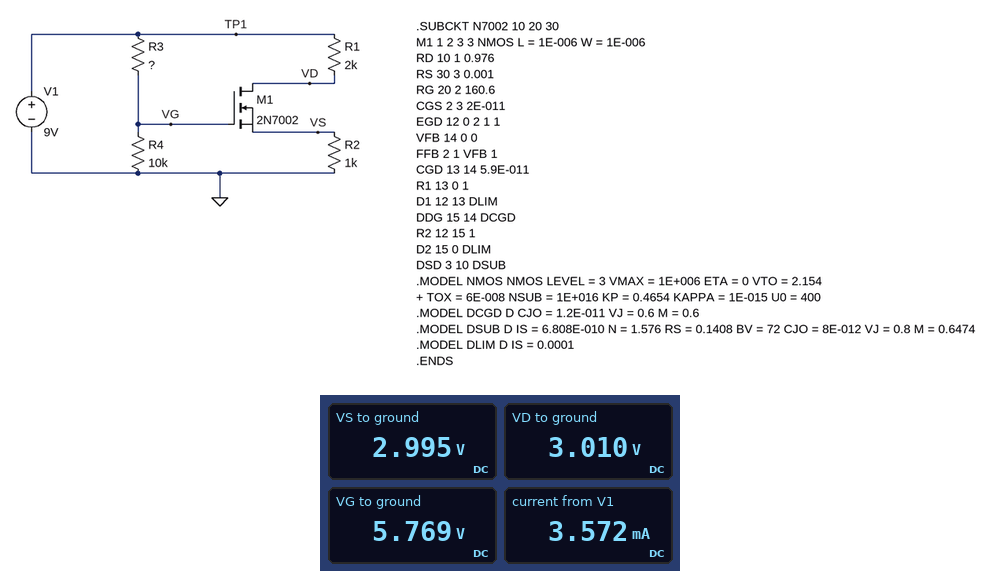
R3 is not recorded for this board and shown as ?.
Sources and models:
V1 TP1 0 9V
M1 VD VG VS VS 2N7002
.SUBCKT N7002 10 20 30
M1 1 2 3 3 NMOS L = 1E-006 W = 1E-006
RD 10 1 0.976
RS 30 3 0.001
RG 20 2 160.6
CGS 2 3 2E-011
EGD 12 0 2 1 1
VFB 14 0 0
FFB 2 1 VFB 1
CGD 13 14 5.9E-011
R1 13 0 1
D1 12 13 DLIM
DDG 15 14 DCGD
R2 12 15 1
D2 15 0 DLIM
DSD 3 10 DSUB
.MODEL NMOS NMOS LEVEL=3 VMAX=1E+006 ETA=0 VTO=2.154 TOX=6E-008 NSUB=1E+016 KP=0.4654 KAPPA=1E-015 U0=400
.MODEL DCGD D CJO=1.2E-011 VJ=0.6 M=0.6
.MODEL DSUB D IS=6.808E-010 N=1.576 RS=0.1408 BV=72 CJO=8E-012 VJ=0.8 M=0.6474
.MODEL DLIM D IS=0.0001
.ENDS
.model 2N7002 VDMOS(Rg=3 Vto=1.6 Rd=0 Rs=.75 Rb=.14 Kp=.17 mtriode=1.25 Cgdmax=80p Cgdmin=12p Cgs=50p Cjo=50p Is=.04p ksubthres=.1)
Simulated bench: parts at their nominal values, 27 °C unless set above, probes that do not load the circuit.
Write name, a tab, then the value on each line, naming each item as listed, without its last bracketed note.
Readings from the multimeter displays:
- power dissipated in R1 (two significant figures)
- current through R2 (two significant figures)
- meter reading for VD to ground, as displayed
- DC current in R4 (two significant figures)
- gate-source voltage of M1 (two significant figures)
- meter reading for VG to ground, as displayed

power dissipated in R1	18 mW
current through R2	3.0 mA
meter reading for VD to ground, as displayed	3.010 V
DC current in R4	580 µA
gate-source voltage of M1	2.8 V
meter reading for VG to ground, as displayed	5.769 V
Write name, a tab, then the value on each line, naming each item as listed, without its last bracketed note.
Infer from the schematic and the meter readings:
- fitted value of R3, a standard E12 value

fitted value of R3, a standard E12 value	5.6 kΩ
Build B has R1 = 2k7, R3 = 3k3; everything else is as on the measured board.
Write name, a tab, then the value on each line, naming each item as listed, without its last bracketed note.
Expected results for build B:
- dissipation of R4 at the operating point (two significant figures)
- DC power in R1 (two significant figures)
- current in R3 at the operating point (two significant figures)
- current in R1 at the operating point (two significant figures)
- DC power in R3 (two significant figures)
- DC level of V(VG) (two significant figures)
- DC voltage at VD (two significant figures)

dissipation of R4 at the operating point	4.6 mW
DC power in R1	16 mW
current in R3 at the operating point	680 µA
current in R1 at the operating point	2.4 mA
DC power in R3	1.5 mW
DC level of V(VG)	6.8 V
DC voltage at VD	2.4 V
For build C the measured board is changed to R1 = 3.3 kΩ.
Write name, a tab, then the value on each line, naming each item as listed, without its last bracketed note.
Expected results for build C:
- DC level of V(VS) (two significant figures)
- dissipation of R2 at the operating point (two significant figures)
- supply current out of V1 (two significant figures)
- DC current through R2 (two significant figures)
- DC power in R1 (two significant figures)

DC level of V(VS)	2.1 V
dissipation of R2 at the operating point	4.4 mW
supply current out of V1	2.7 mA
DC current through R2	2.1 mA
DC power in R1	14 mW
